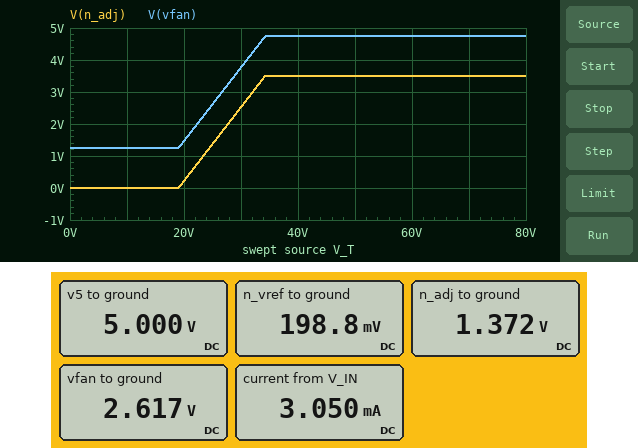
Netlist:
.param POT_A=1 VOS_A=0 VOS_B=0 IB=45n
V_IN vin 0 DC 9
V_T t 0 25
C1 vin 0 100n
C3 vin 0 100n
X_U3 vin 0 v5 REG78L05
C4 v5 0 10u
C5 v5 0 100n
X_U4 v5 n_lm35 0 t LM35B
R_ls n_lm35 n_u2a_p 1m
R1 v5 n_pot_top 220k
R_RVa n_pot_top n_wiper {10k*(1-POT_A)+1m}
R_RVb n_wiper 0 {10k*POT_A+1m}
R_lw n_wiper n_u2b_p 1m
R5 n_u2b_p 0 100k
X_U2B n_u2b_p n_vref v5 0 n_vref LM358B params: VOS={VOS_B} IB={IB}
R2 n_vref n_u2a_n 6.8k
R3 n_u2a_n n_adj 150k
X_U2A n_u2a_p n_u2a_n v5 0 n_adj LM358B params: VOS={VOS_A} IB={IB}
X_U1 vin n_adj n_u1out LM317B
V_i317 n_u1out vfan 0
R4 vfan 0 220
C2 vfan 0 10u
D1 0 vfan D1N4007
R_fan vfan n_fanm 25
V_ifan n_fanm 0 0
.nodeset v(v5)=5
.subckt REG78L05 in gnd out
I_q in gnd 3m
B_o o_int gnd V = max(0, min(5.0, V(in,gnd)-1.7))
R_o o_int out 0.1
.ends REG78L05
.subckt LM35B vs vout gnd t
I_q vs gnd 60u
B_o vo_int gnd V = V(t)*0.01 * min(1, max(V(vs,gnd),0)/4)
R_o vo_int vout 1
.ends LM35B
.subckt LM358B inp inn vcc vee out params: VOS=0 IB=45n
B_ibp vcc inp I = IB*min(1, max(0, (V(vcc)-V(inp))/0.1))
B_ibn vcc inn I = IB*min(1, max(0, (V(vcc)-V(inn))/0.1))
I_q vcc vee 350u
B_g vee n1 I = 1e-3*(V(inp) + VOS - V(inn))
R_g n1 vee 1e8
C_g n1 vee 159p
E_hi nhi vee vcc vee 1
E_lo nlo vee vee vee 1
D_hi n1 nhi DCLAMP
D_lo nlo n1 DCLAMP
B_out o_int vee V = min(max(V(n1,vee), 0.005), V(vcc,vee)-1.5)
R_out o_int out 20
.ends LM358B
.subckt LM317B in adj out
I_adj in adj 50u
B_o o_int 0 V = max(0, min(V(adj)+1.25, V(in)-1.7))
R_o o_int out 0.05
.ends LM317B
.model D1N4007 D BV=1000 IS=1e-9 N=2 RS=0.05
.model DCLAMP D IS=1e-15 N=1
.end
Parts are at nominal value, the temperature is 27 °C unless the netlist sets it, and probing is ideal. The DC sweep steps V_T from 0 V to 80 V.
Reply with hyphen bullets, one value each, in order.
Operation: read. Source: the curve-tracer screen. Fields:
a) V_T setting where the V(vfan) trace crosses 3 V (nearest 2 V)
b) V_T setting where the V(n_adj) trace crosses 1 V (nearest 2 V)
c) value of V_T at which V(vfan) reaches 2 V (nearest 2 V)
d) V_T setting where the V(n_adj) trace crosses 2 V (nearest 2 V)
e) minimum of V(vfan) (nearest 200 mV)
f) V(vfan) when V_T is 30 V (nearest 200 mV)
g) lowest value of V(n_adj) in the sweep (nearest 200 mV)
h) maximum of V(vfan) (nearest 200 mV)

- 26 V
- 24 V
- 22 V
- 28 V
- 1.2 V
- 3.8 V
- 0 V
- 4.8 V
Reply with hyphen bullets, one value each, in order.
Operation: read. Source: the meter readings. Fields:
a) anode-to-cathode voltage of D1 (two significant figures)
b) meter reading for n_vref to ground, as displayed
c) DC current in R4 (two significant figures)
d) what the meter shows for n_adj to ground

- -2.6 V
- 198.8 mV
- 12 mA
- 1.372 V
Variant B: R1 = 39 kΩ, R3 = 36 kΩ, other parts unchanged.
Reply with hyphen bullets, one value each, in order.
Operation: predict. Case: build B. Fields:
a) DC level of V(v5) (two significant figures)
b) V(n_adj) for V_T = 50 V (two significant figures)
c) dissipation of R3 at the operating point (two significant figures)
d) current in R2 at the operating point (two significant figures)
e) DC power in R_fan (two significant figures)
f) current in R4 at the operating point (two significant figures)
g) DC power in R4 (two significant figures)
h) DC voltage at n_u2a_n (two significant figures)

- 5.0 V
- 6.4 mV
- 17 µW
- 22 µA
- 63 mW
- 5.7 mA
- 7.1 mW
- 800 mV
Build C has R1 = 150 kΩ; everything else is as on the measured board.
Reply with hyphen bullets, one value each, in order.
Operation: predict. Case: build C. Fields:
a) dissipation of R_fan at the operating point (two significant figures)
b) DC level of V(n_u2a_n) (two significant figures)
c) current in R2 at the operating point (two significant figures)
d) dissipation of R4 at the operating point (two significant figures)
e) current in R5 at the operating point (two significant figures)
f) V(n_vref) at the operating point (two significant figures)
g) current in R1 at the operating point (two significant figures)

- 63 mW
- 270 mV
- 1.7 µA
- 7.1 mW
- 2.9 µA
- 290 mV
- 31 µA
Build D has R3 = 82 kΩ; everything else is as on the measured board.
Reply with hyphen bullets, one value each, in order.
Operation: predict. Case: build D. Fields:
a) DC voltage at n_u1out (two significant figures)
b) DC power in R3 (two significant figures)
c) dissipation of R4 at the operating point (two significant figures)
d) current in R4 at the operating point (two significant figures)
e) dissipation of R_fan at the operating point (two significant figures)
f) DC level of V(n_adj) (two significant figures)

- 2.1 V
- 4.6 µW
- 20 mW
- 9.6 mA
- 180 mW
- 860 mV
